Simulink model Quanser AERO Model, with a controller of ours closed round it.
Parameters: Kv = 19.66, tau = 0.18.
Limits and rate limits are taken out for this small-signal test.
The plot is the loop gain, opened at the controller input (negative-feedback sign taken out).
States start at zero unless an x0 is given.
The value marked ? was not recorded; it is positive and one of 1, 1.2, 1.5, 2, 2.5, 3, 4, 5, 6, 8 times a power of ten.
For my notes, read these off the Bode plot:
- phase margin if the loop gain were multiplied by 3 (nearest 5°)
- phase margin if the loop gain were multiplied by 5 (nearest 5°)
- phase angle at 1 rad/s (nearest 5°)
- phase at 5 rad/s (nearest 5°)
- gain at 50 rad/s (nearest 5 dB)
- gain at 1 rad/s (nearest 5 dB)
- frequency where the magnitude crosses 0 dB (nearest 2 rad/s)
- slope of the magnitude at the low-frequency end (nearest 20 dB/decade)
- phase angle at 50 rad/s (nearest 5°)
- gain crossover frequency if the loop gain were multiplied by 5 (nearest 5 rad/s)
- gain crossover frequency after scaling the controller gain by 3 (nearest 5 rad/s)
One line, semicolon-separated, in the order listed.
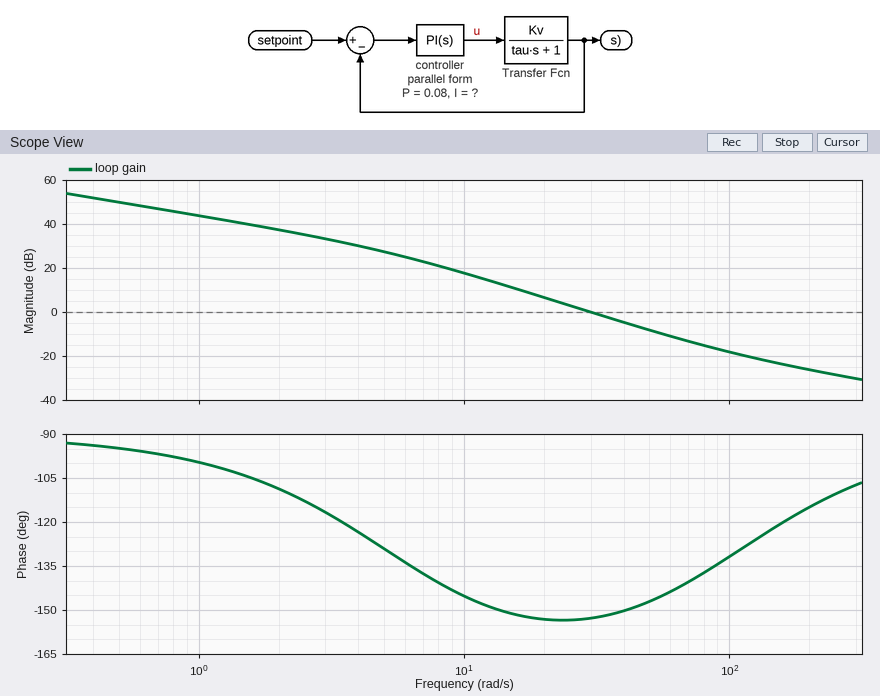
35°; 40°; -100°; -130°; -10 dB; 45 dB; 30 rad/s; -20 dB/decade; -145°; 75 rad/s; 55 rad/s
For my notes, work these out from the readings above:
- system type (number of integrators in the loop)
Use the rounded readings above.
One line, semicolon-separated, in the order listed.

1
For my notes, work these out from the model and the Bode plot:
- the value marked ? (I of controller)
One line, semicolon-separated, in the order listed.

8
